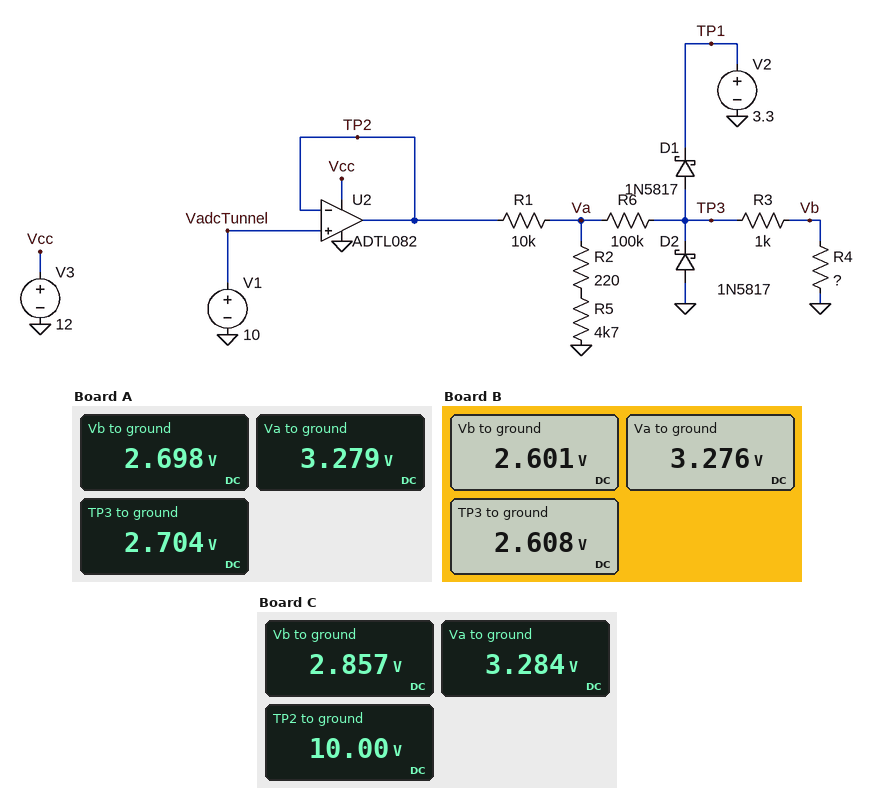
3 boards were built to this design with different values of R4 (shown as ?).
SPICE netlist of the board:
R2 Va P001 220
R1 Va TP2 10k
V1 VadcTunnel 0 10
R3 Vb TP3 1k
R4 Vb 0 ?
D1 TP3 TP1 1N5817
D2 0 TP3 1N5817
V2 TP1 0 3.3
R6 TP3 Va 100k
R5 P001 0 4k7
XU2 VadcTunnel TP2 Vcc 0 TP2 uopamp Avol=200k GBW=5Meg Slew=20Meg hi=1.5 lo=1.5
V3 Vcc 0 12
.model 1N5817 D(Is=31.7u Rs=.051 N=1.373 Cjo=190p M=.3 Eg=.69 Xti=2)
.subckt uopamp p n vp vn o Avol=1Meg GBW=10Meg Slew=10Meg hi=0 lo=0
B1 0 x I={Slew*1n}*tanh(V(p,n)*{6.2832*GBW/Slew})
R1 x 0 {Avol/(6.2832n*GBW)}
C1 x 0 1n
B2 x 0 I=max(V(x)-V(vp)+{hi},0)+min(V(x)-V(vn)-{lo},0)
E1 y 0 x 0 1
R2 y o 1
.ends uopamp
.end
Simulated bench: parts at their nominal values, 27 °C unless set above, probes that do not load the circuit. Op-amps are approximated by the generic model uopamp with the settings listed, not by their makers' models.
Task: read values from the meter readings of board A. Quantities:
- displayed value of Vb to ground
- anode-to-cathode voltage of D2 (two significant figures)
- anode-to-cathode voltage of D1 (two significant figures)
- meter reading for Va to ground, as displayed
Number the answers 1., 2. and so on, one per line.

1. 2.698 V
2. -2.7 V
3. -600 mV
4. 3.279 V
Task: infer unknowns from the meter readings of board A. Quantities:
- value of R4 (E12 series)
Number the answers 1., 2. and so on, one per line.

1. 470 kΩ
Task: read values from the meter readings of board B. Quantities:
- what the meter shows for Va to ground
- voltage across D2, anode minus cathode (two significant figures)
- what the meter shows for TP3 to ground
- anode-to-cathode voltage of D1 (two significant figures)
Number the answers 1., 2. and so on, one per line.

1. 3.276 V
2. -2.6 V
3. 2.608 V
4. -690 mV
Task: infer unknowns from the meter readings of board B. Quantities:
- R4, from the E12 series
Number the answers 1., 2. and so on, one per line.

1. 390 kΩ
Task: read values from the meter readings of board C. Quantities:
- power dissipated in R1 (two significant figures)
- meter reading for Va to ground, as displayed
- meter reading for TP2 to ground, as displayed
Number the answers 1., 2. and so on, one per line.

1. 4.5 mW
2. 3.284 V
3. 10.00 V
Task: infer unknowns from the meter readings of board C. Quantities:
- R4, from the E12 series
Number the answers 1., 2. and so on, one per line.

1. 680 kΩ
